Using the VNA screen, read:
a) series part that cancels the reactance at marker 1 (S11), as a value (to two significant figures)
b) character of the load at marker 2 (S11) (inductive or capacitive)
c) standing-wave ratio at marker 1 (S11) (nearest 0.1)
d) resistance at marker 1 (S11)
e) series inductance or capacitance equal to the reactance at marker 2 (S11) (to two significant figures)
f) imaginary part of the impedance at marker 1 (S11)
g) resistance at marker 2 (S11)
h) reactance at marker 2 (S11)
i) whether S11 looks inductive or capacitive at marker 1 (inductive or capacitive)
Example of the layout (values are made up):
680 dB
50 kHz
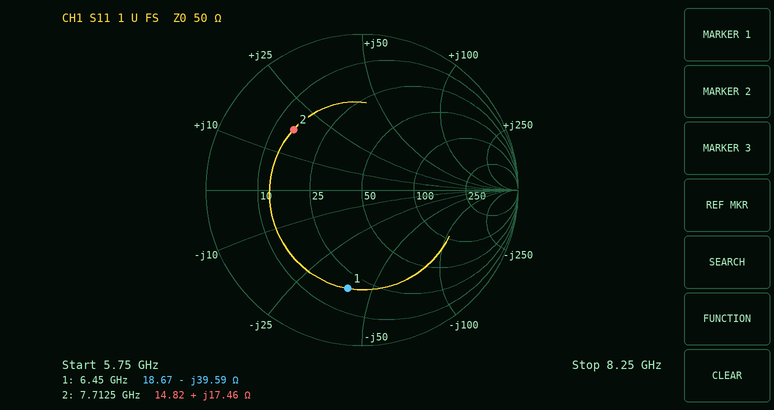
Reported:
980 pH
inductive
4.5
18.67 Ω
360 pH
-39.59 Ω
14.82 Ω
+17.46 Ω
capacitive
